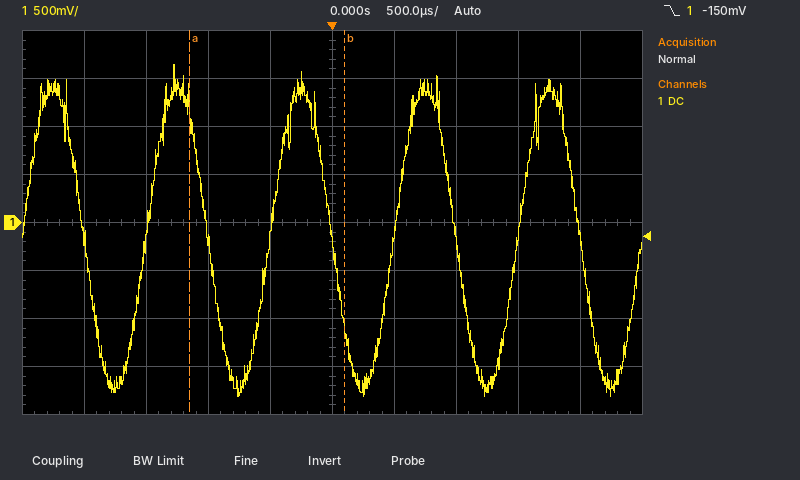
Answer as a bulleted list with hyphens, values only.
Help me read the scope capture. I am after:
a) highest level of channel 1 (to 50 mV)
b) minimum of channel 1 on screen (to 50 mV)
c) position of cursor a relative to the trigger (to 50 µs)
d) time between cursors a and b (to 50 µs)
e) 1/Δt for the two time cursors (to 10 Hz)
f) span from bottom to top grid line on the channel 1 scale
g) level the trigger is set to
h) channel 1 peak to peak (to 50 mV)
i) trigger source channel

- 1.65 V
- -1.80 V
- -1.15 ms
- 1.25 ms
- 800 Hz
- 4 V
- -150 mV
- 3.45 V
- channel 1
